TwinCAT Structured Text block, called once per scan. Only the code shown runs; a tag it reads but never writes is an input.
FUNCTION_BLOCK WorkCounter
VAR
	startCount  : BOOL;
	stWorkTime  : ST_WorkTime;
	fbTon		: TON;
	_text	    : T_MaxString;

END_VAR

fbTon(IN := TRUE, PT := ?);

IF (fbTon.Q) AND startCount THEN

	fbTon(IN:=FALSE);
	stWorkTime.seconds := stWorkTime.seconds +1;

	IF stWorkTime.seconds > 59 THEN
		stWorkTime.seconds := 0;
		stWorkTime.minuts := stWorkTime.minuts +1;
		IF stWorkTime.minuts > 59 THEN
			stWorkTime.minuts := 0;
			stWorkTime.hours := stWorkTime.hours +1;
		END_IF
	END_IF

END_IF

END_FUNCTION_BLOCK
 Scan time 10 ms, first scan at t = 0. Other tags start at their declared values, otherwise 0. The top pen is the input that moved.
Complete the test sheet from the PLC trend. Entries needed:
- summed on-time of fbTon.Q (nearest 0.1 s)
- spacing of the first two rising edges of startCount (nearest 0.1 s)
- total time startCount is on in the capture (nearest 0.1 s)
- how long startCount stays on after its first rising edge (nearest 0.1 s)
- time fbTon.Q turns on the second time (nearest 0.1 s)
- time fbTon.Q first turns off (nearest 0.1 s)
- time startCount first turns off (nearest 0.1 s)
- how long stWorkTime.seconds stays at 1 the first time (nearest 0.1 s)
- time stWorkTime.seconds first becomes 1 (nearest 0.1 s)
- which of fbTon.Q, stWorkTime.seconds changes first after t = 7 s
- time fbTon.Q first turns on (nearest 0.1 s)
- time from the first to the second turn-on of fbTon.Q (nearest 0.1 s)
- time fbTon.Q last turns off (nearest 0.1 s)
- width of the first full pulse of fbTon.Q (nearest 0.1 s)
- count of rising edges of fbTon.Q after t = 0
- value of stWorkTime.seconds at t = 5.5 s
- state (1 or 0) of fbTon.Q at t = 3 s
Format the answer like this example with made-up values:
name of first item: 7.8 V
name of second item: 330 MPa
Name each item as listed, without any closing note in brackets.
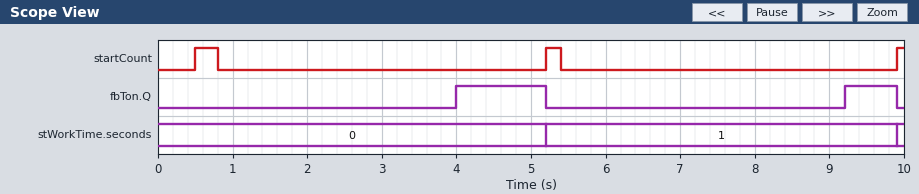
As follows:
summed on-time of fbTon.Q: 1.9 s
spacing of the first two rising edges of startCount: 4.7 s
total time startCount is on in the capture: 0.6 s
how long startCount stays on after its first rising edge: 0.3 s
time fbTon.Q turns on the second time: 9.2 s
time fbTon.Q first turns off: 5.2 s
time startCount first turns off: 0.8 s
how long stWorkTime.seconds stays at 1 the first time: 4.7 s
time stWorkTime.seconds first becomes 1: 5.2 s
which of fbTon.Q, stWorkTime.seconds changes first after t = 7 s: fbTon.Q
time fbTon.Q first turns on: 4.0 s
time from the first to the second turn-on of fbTon.Q: 5.2 s
time fbTon.Q last turns off: 9.9 s
width of the first full pulse of fbTon.Q: 1.2 s
count of rising edges of fbTon.Q after t = 0: 2
value of stWorkTime.seconds at t = 5.5 s: 1
state (1 or 0) of fbTon.Q at t = 3 s: 0
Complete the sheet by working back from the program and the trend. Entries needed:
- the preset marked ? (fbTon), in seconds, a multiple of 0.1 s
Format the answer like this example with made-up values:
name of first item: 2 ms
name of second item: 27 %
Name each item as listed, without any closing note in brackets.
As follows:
the preset marked ? (fbTon), in seconds, a multiple of 0.1 s: 4.0 s
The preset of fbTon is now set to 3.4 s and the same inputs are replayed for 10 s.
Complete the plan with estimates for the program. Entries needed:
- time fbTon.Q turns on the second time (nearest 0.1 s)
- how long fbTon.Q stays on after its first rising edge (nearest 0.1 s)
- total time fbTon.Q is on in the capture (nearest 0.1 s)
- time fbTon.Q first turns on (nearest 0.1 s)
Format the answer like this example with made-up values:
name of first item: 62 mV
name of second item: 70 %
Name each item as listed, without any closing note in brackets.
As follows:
time fbTon.Q turns on the second time: 8.6 s
how long fbTon.Q stays on after its first rising edge: 1.8 s
total time fbTon.Q is on in the capture: 3.1 s
time fbTon.Q first turns on: 3.4 s
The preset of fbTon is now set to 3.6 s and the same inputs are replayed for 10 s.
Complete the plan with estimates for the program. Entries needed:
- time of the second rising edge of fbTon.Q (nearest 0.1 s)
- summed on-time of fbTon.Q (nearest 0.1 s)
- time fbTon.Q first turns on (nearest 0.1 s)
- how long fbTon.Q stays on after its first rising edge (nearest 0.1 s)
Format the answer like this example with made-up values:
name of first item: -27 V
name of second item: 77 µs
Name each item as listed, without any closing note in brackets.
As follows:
time of the second rising edge of fbTon.Q: 8.8 s
summed on-time of fbTon.Q: 2.7 s
time fbTon.Q first turns on: 3.6 s
how long fbTon.Q stays on after its first rising edge: 1.6 s
